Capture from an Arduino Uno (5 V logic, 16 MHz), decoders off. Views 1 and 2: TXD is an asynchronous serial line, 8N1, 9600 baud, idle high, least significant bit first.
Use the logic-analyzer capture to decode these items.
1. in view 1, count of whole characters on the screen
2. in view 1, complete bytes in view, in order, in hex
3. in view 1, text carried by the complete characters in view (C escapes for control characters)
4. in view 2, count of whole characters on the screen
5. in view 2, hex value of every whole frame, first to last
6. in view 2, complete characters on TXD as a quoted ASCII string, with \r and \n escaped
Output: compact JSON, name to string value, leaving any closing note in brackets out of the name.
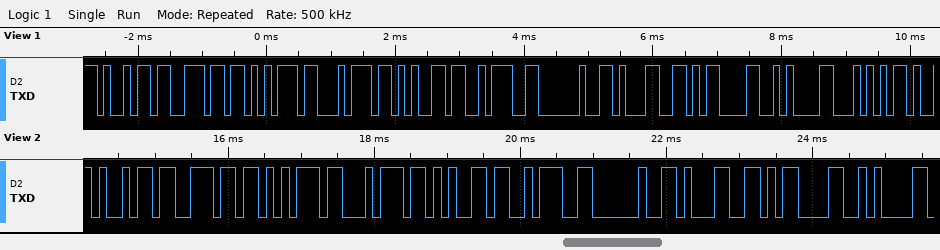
{"in view 1, count of whole characters on the screen": "11", "in view 1, complete bytes in view, in order, in hex": "69 6E 75 74 65 3A 20 31 0D 0A 54", "in view 1, text carried by the complete characters in view": "\"inute: 1\\r\\nT\"", "in view 2, count of whole characters on the screen": "10", "in view 2, hex value of every whole frame, first to last": "69 6E 75 74 65 3A 20 31 0D 0A", "in view 2, complete characters on TXD as a quoted ASCII string, with \\r and \\n escaped": "\"inute: 1\\r\\n\""}
